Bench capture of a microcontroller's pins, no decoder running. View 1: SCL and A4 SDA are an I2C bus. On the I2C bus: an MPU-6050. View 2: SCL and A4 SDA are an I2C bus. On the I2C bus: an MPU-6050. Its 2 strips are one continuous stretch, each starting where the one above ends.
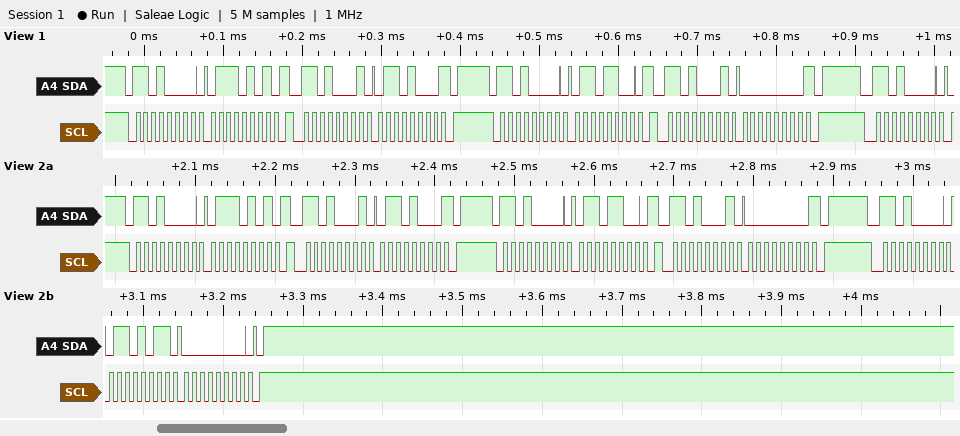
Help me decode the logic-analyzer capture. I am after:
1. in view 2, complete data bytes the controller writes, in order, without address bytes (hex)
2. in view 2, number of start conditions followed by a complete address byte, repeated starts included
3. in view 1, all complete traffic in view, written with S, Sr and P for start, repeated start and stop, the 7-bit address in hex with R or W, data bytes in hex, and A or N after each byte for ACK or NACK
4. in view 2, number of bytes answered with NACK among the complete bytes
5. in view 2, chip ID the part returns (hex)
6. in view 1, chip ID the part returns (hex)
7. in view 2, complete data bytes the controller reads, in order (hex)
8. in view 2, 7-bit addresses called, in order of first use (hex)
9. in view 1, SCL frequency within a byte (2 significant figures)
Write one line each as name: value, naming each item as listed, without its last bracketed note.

in view 2, complete data bytes the controller writes, in order, without address bytes: 75 6C 6B 00
in view 2, number of start conditions followed by a complete address byte, repeated starts included: 5
in view 1, all complete traffic in view, written with S, Sr and P for start, repeated start and stop, the 7-bit address in hex with R or W, data bytes in hex, and A or N after each byte for ACK or NACK: S 68W A 75 A Sr 68R A 68 N P S 68W A 6C A Sr 68R A 00 N P S 68W A
in view 2, number of bytes answered with NACK among the complete bytes: 2
in view 2, chip ID the part returns: 0x68
in view 1, chip ID the part returns: 0x68
in view 2, complete data bytes the controller reads, in order: 68 00
in view 2, 7-bit addresses called, in order of first use: 0x68
in view 1, SCL frequency within a byte: 100 kHz
